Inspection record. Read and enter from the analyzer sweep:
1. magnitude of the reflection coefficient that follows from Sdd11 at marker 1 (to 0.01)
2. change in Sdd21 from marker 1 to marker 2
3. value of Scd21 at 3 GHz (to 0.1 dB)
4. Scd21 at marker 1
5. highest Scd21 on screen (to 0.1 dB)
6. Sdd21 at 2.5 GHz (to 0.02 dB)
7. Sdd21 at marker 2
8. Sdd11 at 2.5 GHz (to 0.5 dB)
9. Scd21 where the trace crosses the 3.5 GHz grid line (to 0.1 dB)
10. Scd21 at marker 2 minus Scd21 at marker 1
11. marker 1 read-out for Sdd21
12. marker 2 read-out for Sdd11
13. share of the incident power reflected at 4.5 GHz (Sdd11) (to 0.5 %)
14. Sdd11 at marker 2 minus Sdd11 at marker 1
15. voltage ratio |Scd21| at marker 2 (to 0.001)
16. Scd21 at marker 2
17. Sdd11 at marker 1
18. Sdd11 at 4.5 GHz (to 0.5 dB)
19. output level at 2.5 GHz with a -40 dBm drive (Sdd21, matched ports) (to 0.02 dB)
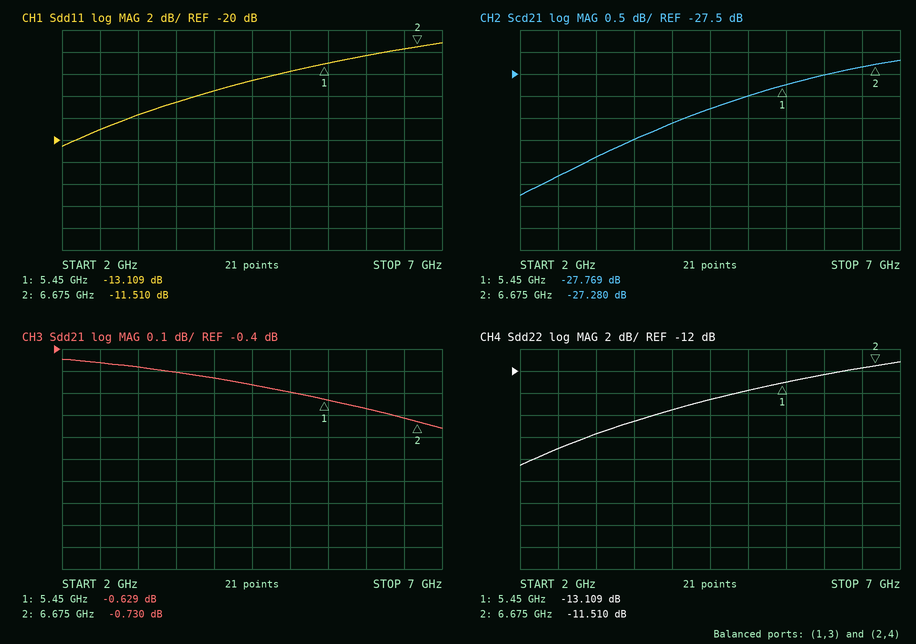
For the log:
0.22
-0.101 dB
-29.4 dB
-27.769 dB
-27.2 dB
-0.46 dB
-0.730 dB
-19.0 dB
-29.0 dB
0.489 dB
-0.629 dB
-11.510 dB
3.5 %
1.599 dB
0.043
-27.280 dB
-13.109 dB
-14.5 dB
-40.46 dBm
